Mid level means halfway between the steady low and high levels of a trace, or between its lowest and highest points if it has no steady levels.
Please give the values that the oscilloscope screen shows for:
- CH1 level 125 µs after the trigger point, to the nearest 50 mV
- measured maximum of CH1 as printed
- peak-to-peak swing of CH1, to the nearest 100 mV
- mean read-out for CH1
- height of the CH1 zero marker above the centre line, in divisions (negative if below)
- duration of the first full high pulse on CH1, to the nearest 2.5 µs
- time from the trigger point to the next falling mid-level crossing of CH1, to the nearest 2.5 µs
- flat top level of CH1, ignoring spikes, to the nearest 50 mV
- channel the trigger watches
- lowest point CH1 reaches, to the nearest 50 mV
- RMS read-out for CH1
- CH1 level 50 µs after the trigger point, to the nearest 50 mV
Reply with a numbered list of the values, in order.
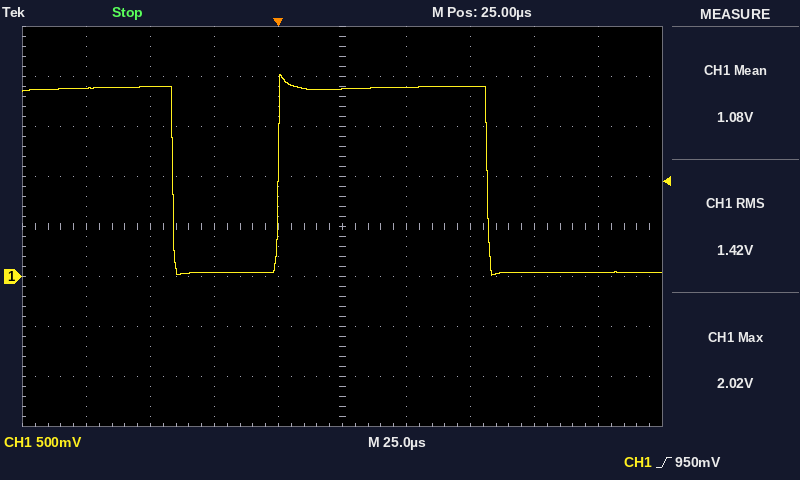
1. 50 mV
2. 2.02 V
3. 2.00 V
4. 1.08 V
5. -1.0 div
6. 82.5 µs
7. 82.5 µs
8. 1.90 V
9. CH1
10. 0 mV
11. 1.42 V
12. 1.90 V
